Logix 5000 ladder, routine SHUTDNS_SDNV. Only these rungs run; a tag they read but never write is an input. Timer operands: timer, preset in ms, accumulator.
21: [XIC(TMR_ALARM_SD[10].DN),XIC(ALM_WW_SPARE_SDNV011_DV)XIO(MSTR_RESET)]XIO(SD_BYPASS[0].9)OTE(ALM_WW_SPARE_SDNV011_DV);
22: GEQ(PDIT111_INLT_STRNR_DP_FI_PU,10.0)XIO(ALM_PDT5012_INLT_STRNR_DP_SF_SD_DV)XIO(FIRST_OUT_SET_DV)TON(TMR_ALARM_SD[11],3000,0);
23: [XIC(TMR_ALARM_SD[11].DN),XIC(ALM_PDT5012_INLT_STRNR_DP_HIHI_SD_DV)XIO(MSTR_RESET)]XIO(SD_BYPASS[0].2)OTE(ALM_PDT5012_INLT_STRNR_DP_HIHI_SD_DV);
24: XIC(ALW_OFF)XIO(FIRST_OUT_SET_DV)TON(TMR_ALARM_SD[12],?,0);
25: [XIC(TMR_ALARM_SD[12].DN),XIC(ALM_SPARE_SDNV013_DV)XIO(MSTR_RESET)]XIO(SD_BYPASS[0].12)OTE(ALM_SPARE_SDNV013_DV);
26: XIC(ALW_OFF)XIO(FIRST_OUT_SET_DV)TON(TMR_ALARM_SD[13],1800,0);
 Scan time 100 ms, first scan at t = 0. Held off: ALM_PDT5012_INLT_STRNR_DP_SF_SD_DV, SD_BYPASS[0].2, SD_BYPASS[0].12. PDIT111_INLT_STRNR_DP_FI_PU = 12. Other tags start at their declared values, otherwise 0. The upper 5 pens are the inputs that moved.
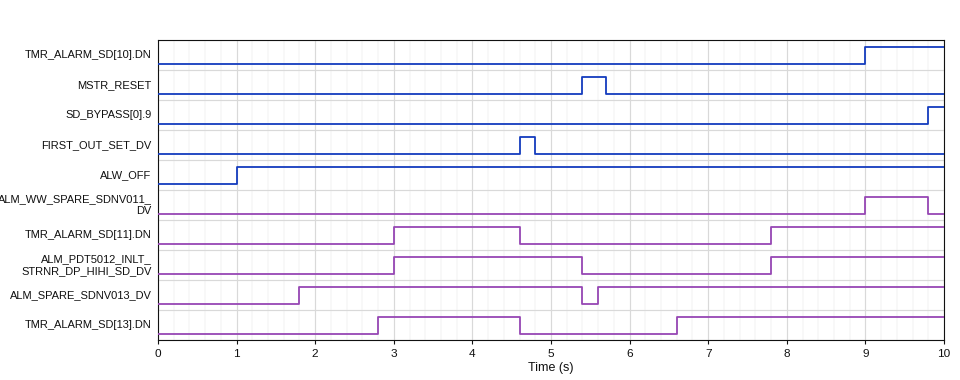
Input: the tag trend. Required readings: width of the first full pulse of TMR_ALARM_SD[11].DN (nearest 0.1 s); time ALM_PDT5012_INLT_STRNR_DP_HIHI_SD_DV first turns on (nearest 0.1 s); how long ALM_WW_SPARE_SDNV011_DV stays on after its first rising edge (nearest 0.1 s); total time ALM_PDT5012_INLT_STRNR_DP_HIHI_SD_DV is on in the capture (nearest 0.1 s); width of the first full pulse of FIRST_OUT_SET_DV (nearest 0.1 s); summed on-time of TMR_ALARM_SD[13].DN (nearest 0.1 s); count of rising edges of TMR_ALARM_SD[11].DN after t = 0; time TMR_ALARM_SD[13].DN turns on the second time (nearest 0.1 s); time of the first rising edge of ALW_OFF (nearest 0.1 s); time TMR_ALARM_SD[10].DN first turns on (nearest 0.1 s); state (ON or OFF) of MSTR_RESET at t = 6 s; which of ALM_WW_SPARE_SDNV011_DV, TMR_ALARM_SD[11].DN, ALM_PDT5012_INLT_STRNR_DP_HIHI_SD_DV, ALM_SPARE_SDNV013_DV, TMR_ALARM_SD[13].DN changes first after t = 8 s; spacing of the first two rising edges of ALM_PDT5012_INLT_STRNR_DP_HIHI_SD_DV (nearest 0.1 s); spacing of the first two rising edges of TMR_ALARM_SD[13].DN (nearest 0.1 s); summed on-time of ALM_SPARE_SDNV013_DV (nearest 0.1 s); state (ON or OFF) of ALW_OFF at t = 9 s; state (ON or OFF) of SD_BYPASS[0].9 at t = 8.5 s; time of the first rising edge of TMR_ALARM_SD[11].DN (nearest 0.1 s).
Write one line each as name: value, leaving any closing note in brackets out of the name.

width of the first full pulse of TMR_ALARM_SD[11].DN: 1.6 s
time ALM_PDT5012_INLT_STRNR_DP_HIHI_SD_DV first turns on: 3.0 s
how long ALM_WW_SPARE_SDNV011_DV stays on after its first rising edge: 0.8 s
total time ALM_PDT5012_INLT_STRNR_DP_HIHI_SD_DV is on in the capture: 4.6 s
width of the first full pulse of FIRST_OUT_SET_DV: 0.2 s
summed on-time of TMR_ALARM_SD[13].DN: 5.2 s
count of rising edges of TMR_ALARM_SD[11].DN after t = 0: 2
time TMR_ALARM_SD[13].DN turns on the second time: 6.6 s
time of the first rising edge of ALW_OFF: 1.0 s
time TMR_ALARM_SD[10].DN first turns on: 9.0 s
state (ON or OFF) of MSTR_RESET at t = 6 s: OFF
which of ALM_WW_SPARE_SDNV011_DV, TMR_ALARM_SD[11].DN, ALM_PDT5012_INLT_STRNR_DP_HIHI_SD_DV, ALM_SPARE_SDNV013_DV, TMR_ALARM_SD[13].DN changes first after t = 8 s: ALM_WW_SPARE_SDNV011_DV
spacing of the first two rising edges of ALM_PDT5012_INLT_STRNR_DP_HIHI_SD_DV: 4.8 s
spacing of the first two rising edges of TMR_ALARM_SD[13].DN: 3.8 s
summed on-time of ALM_SPARE_SDNV013_DV: 8.0 s
state (ON or OFF) of ALW_OFF at t = 9 s: ON
state (ON or OFF) of SD_BYPASS[0].9 at t = 8.5 s: OFF
time of the first rising edge of TMR_ALARM_SD[11].DN: 3.0 s
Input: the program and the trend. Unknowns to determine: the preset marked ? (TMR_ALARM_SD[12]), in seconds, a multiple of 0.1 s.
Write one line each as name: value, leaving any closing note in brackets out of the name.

the preset marked ? (TMR_ALARM_SD[12]), in seconds, a multiple of 0.1 s: 0.8 s
